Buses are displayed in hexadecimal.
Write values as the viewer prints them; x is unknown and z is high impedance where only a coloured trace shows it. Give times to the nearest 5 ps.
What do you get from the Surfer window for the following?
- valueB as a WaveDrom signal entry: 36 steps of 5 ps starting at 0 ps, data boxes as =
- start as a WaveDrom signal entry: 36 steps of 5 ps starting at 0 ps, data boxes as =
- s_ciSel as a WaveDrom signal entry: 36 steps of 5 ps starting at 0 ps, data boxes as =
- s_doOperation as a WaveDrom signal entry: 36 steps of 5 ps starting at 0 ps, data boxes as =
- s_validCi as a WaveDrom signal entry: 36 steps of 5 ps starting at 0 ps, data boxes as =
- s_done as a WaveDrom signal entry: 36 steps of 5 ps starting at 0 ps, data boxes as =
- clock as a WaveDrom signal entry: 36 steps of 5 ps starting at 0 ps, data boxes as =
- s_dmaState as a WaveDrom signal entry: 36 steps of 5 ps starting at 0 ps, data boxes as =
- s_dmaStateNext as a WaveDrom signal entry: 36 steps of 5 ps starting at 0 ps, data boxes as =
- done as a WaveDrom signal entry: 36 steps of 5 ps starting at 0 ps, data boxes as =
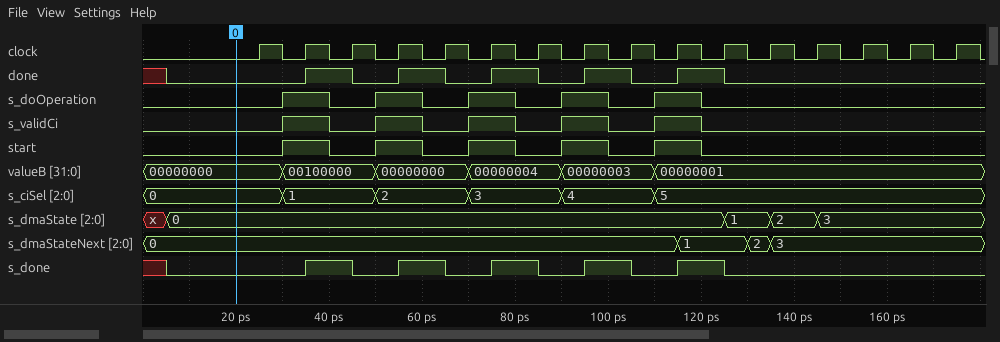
{name: 'valueB', wave: '=.....=...=...=...=...=.............', data: '00000000 00100000 00000000 00000004 00000003 00000001'}
{name: 'start', wave: '0.....1.0.1.0.1.0.1.0.1.0...........'}
{name: 's_ciSel', wave: '=.....=...=...=...=...=.............', data: '0 1 2 3 4 5'}
{name: 's_doOperation', wave: '0.....1.0.1.0.1.0.1.0.1.0...........'}
{name: 's_validCi', wave: '0.....1.0.1.0.1.0.1.0.1.0...........'}
{name: 's_done', wave: 'x0.....1.0.1.0.1.0.1.0.1.0..........'}
{name: 'clock', wave: '0....1010101010101010101010101010101'}
{name: 's_dmaState', wave: 'x=.......................=.=.=......', data: '0 1 2 3'}
{name: 's_dmaStateNext', wave: '=......................=..==........', data: '0 1 2 3'}
{name: 'done', wave: 'x0.....1.0.1.0.1.0.1.0.1.0..........'}
